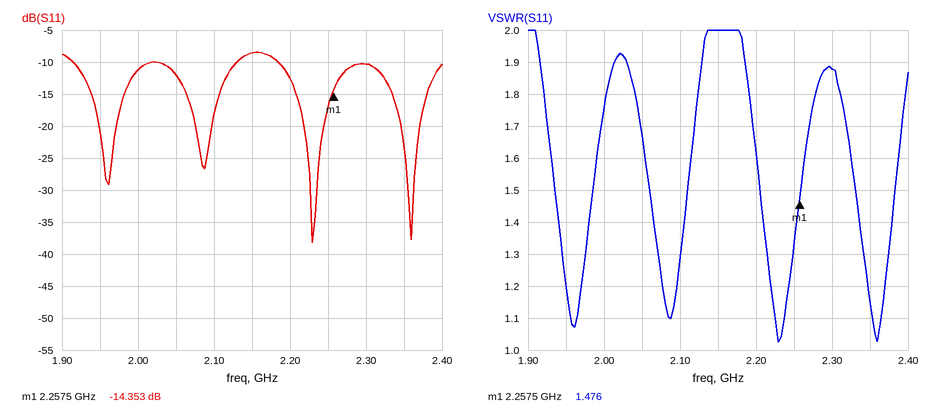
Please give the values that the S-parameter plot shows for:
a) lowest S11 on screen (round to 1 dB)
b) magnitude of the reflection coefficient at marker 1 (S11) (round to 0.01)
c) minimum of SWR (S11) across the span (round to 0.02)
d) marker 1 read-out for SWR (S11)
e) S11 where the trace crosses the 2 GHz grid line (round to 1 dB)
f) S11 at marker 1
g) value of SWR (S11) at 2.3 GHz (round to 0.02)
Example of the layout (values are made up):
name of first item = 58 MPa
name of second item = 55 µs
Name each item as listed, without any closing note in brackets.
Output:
lowest S11 on screen = -38 dB
magnitude of the reflection coefficient at marker 1 (S11) = 0.19
minimum of SWR (S11) across the span = 1.02
marker 1 read-out for SWR = 1.476
S11 where the trace crosses the 2 GHz grid line = -11 dB
S11 at marker 1 = -14.353 dB
value of SWR (S11) at 2.3 GHz = 1.88
